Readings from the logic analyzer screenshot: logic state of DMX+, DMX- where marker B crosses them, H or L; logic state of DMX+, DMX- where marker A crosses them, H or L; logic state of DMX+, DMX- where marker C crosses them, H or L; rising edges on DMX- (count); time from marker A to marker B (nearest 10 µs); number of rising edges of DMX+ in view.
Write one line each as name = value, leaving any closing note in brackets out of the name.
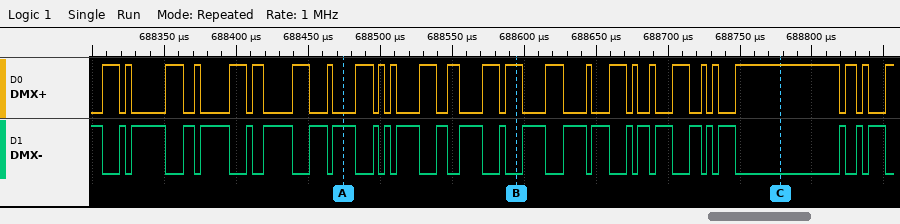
logic state of DMX+, DMX- where marker B crosses them, H or L = DMX+=H, DMX-=L
logic state of DMX+, DMX- where marker A crosses them, H or L = DMX+=L, DMX-=H
logic state of DMX+, DMX- where marker C crosses them, H or L = DMX+=H, DMX-=L
rising edges on DMX- = 26
time from marker A to marker B = 120 µs
number of rising edges of DMX+ in view = 27
